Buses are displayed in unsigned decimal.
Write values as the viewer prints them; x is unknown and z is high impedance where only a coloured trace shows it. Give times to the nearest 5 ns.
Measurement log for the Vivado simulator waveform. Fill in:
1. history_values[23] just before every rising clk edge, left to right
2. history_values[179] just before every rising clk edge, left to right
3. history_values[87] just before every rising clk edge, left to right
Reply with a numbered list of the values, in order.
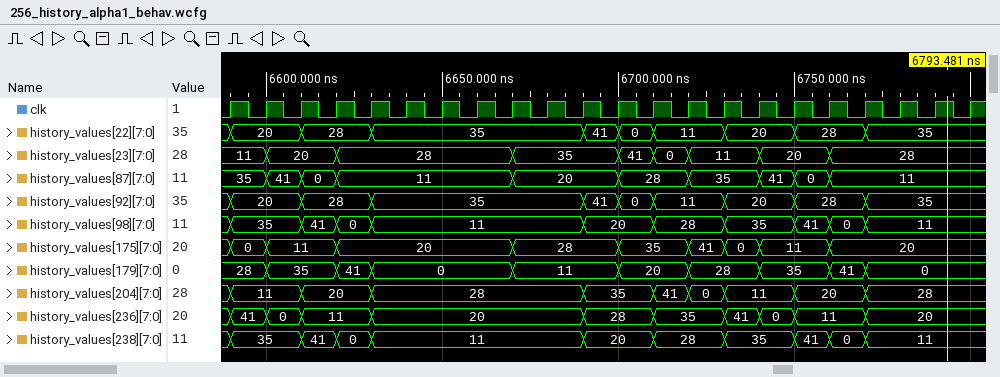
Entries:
1. 11, 11, 20, 20, 28, 28, 28, 28, 28, 35, 35, 35, 41, 0, 11, 11, 20, 20, 28, 28, 28, 28
2. 28, 28, 35, 35, 41, 0, 0, 0, 0, 11, 11, 11, 20, 20, 28, 28, 35, 35, 41, 0, 0, 0
3. 35, 35, 41, 0, 11, 11, 11, 11, 11, 20, 20, 20, 28, 28, 35, 35, 41, 0, 11, 11, 11, 11
